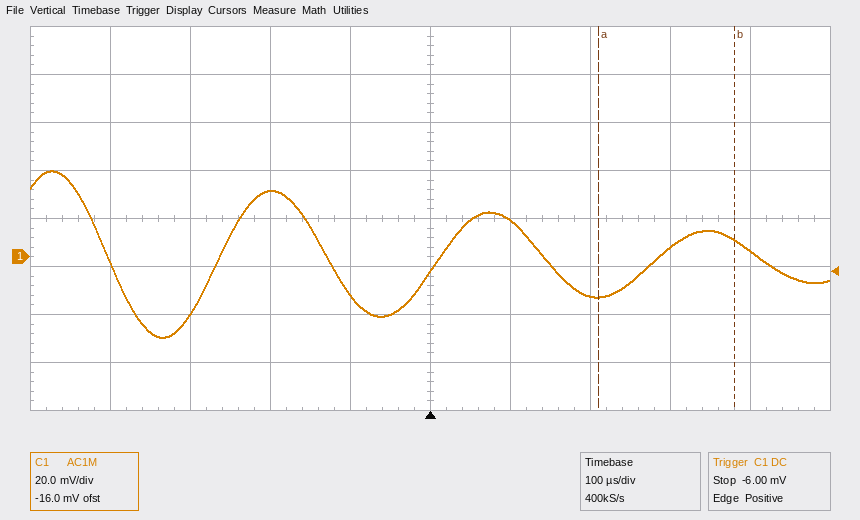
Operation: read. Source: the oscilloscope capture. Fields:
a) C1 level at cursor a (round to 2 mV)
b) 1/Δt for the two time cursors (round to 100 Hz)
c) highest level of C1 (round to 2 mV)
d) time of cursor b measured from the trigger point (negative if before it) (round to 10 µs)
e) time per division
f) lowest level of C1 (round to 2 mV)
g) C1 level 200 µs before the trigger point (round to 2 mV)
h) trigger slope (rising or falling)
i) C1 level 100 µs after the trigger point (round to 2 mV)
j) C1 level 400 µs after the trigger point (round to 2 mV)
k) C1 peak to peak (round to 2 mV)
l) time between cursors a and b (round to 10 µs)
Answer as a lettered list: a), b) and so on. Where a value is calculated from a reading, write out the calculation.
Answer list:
a) -16 mV
b) 1 / 170 µs ≈ 5.9 kHz
c) 36 mV
d) +380 µs
e) 100 µs
f) -34 mV
g) 28 mV
h) rising
i) 16 mV
j) 2 mV
k) 36 mV − (-34 mV) = 70 mV
l) 170 µs
